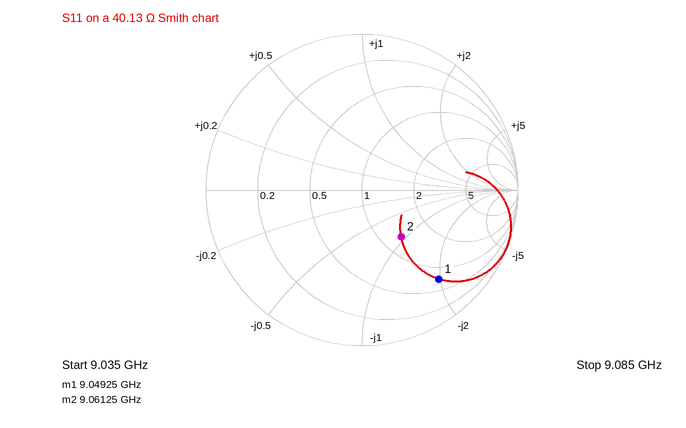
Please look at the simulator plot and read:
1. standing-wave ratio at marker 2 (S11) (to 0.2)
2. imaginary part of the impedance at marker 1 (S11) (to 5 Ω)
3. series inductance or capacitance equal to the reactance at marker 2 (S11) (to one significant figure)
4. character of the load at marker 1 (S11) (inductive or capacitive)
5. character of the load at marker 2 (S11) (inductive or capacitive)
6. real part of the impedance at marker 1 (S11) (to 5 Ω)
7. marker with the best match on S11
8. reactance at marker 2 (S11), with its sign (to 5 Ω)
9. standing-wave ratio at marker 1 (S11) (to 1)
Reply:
2.2
-80 Ω
500 fF
capacitive
capacitive
30 Ω
marker 2
-35 Ω
7
